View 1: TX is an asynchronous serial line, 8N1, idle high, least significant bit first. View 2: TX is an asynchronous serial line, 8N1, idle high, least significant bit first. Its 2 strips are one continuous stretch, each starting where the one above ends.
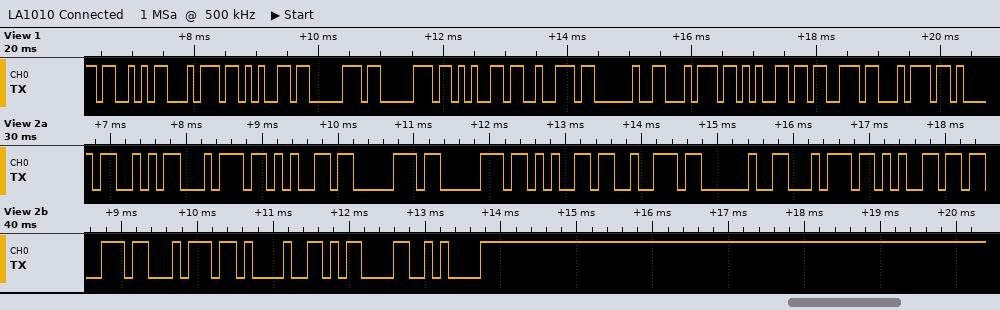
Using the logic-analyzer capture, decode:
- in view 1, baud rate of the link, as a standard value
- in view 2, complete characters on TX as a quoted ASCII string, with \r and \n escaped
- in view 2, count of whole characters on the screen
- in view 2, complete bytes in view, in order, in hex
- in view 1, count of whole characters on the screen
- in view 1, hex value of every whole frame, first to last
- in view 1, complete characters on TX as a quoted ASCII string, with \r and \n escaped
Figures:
9600 baud
"Stepper test!\r\n"
15
53 74 65 70 70 65 72 20 74 65 73 74 21 0D 0A
12
53 74 65 70 70 65 72 20 74 65 73 74
"Stepper test"
